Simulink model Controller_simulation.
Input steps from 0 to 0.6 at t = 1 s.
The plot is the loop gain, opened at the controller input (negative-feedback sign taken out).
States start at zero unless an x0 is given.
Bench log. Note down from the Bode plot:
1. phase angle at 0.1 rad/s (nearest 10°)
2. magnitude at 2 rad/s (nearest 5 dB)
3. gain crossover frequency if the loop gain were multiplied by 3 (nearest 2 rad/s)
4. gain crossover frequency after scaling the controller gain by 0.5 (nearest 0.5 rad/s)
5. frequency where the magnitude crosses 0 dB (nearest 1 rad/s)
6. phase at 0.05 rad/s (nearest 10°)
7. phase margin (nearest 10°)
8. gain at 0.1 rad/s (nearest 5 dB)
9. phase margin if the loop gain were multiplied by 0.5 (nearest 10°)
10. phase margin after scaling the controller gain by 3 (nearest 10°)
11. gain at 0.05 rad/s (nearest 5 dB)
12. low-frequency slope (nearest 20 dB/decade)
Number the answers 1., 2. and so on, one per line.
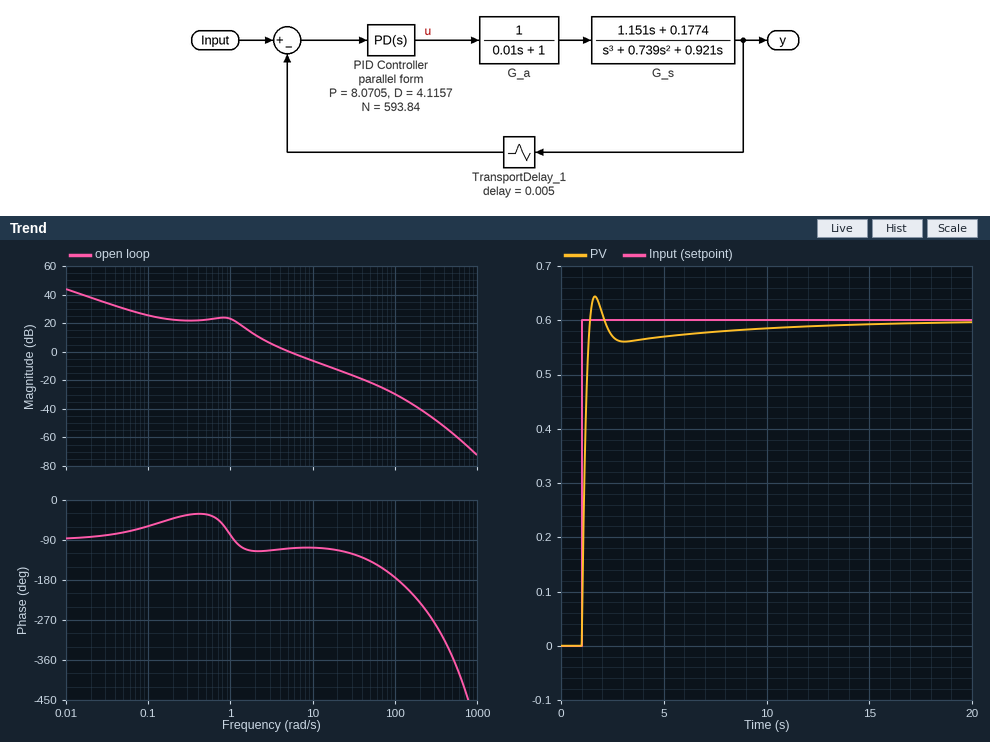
1. -60°
2. 10 dB
3. 14 rad/s
4. 3.0 rad/s
5. 5 rad/s
6. -70°
7. 70°
8. 25 dB
9. 70°
10. 70°
11. 30 dB
12. -20 dB/decade
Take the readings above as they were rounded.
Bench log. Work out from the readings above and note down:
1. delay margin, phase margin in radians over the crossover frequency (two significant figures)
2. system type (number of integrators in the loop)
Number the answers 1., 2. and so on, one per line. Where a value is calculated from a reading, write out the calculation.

1. 70 × π / 180 / 5 = 0.24 s
2. 1
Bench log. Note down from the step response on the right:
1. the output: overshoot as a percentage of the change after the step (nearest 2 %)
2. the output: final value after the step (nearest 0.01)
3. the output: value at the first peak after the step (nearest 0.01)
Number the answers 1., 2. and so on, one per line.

1. 8 %
2. 0.60
3. 0.64
